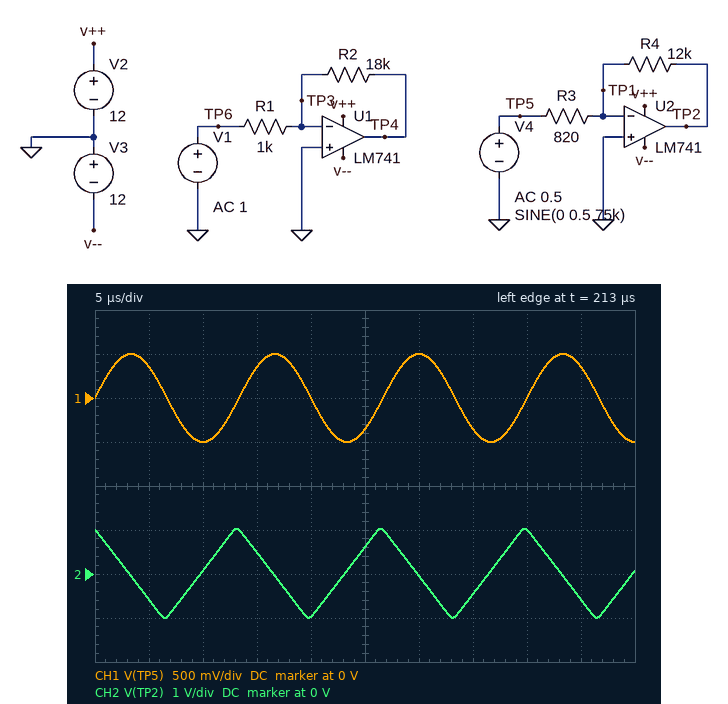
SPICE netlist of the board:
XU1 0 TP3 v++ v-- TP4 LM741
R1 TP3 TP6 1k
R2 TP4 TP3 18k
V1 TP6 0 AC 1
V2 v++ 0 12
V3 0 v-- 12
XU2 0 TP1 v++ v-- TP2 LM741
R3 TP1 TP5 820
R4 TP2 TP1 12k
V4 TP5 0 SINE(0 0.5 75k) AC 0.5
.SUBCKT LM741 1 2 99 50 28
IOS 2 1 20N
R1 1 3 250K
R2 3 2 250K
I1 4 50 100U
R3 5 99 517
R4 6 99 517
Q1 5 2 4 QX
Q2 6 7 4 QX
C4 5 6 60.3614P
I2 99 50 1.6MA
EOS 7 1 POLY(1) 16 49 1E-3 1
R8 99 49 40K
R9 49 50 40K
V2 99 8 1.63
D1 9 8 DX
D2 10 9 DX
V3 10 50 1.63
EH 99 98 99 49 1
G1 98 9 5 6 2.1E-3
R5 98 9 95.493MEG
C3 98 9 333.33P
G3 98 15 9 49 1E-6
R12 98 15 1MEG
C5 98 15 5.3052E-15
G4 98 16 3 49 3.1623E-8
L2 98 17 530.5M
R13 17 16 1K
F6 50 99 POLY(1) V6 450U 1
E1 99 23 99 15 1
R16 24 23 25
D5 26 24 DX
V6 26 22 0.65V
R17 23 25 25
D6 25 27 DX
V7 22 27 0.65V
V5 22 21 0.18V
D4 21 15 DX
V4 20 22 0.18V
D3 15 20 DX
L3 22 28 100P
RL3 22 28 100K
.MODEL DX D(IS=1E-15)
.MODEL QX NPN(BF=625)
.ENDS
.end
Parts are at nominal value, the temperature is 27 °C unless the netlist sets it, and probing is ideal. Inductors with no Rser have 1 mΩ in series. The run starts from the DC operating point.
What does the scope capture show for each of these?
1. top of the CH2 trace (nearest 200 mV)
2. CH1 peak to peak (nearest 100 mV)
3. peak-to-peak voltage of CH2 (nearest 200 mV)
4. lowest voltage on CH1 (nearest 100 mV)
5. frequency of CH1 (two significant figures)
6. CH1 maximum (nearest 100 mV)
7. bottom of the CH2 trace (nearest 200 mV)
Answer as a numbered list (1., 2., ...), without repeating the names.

1. 1.0 V
2. 1.0 V
3. 2.0 V
4. -500 mV
5. 75 kHz
6. 500 mV
7. -1.0 V
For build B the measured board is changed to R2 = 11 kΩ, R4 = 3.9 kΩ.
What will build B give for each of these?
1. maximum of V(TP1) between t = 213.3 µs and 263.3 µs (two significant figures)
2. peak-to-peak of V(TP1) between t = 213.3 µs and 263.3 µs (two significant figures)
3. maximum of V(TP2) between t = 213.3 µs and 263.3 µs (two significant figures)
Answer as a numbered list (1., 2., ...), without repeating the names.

1. 390 mV
2. 780 mV
3. 990 mV
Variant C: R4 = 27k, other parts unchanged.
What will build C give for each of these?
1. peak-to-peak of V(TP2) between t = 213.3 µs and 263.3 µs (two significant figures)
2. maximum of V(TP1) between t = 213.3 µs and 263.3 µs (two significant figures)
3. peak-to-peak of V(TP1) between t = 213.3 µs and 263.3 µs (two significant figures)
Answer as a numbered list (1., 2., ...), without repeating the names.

1. 2.1 V
2. 480 mV
3. 970 mV
